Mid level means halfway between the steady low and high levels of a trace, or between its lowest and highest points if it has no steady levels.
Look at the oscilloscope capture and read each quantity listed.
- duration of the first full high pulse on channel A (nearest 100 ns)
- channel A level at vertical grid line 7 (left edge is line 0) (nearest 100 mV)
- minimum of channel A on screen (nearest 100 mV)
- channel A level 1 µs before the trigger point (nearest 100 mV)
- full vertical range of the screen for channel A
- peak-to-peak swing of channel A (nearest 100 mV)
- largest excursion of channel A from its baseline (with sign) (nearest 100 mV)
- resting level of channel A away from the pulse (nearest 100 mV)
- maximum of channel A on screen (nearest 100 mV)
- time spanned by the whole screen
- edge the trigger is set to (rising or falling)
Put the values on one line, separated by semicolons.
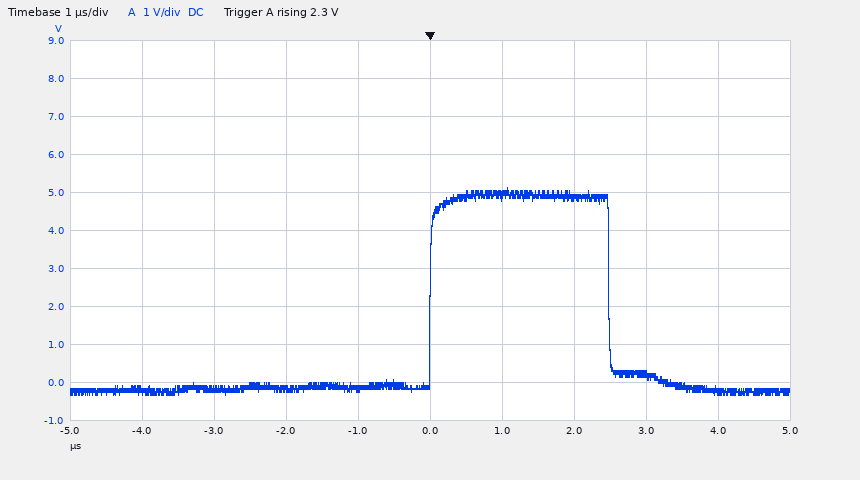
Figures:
2.5 µs; 4.9 V; -300 mV; -200 mV; 10 V; 5.4 V; +5.3 V; -200 mV; 5.1 V; 10 µs; rising
